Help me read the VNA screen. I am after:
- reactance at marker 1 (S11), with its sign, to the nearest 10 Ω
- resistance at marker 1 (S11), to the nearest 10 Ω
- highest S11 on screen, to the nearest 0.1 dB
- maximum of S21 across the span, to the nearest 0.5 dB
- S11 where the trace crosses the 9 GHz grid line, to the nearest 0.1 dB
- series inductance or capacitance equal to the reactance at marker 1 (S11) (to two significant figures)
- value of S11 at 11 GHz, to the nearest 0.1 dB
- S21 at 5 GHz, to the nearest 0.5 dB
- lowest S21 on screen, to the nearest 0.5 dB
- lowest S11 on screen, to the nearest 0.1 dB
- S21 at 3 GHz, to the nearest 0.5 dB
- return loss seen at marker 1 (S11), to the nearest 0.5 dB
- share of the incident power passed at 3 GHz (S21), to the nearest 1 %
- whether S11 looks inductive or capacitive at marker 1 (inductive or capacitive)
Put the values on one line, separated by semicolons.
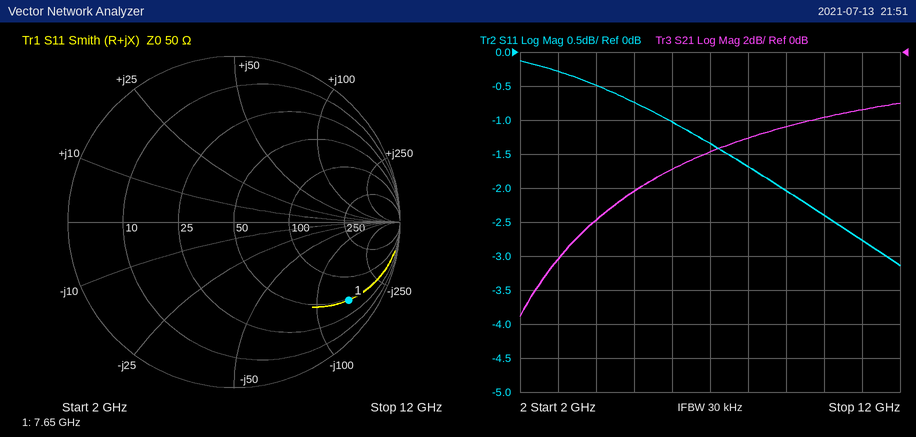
-150 Ω; 50 Ω; -0.1 dB; -3.0 dB; -2.0 dB; 140 fF; -2.8 dB; -8.0 dB; -15.5 dB; -3.1 dB; -12.0 dB; 1.5 dB; 6 %; capacitive
